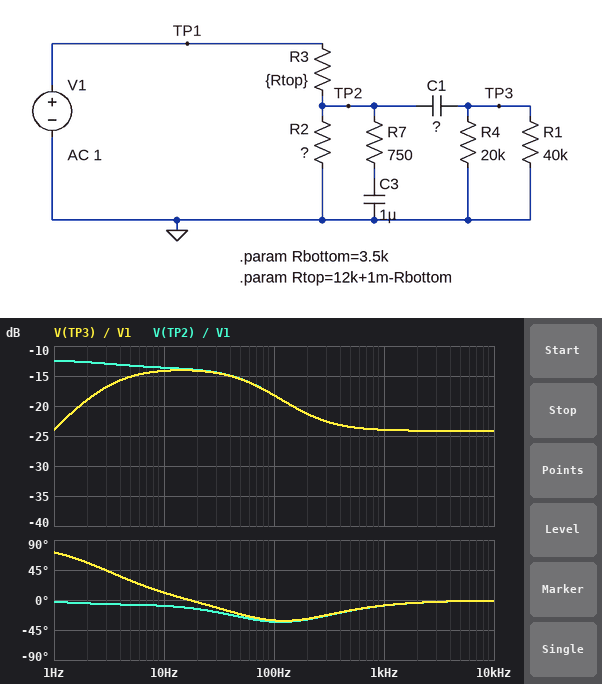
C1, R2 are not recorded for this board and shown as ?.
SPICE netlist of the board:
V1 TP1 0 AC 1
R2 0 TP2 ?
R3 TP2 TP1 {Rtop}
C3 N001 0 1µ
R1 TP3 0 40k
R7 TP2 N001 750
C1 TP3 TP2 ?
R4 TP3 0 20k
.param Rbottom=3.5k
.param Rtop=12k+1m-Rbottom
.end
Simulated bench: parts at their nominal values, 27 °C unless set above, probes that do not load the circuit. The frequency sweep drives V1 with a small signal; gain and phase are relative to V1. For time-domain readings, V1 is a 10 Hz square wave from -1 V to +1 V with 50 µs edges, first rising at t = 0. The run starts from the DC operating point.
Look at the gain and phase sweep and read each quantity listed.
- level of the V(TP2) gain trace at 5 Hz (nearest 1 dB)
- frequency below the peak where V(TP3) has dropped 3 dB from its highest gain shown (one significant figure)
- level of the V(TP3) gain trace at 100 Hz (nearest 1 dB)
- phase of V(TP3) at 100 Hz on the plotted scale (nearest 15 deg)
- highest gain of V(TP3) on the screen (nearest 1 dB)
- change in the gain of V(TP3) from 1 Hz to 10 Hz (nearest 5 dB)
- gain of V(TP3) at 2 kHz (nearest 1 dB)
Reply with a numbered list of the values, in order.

1. -13 dB
2. 3 Hz
3. -18 dB
4. -30 deg
5. -14 dB
6. 10 dB
7. -24 dB
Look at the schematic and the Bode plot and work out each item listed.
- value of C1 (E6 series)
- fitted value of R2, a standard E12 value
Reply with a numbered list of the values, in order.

1. 3.3 µF
2. 2.7 kΩ
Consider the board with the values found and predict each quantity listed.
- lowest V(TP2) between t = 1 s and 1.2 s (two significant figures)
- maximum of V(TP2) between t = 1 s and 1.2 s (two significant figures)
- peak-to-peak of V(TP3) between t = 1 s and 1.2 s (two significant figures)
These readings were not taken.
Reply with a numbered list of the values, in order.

1. -220 mV
2. 220 mV
3. 510 mV
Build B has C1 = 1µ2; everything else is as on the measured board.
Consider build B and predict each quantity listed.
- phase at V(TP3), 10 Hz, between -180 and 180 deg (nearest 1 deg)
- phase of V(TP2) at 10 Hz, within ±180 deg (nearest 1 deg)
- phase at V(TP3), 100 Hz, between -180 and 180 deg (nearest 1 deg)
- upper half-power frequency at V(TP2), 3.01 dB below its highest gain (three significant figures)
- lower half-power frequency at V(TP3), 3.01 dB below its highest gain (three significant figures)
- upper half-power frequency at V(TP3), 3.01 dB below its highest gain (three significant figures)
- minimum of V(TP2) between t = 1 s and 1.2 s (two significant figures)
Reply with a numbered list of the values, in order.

1. 34 deg
2. -11 deg
3. -27 deg
4. 47.2 Hz
5. 6.91 Hz
6. 89.7 Hz
7. -240 mV
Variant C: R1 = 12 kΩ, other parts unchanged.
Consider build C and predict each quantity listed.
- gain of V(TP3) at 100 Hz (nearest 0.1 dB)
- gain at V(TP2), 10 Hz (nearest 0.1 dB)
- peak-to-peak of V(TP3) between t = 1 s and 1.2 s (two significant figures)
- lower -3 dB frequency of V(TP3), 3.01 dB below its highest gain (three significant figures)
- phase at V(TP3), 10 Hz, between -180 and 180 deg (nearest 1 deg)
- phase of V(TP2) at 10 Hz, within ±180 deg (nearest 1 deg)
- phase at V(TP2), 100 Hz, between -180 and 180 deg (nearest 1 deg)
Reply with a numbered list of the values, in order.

1. -18.7 dB
2. -14.1 dB
3. 500 mV
4. 4.41 Hz
5. 21 deg
6. -12 deg
7. -31 deg
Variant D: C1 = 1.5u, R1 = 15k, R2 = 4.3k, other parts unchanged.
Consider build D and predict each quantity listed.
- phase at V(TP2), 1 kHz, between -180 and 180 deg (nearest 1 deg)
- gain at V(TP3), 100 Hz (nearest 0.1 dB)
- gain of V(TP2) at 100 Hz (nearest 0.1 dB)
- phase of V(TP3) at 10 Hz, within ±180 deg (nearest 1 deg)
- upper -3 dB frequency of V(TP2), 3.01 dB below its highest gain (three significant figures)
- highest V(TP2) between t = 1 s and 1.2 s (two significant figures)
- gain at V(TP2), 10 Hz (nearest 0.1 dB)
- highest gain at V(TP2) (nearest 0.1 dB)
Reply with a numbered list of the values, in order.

1. -9 deg
2. -17.6 dB
3. -17.5 dB
4. 34 deg
5. 23.1 Hz
6. 320 mV
7. -11.0 dB
8. -9.5 dB
